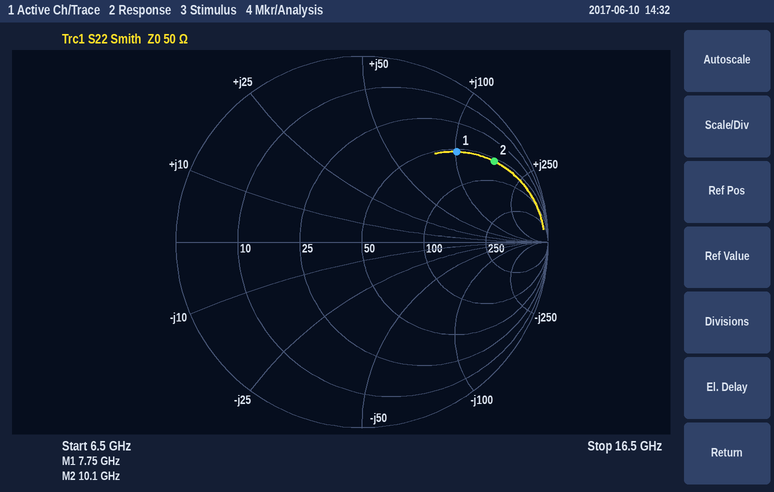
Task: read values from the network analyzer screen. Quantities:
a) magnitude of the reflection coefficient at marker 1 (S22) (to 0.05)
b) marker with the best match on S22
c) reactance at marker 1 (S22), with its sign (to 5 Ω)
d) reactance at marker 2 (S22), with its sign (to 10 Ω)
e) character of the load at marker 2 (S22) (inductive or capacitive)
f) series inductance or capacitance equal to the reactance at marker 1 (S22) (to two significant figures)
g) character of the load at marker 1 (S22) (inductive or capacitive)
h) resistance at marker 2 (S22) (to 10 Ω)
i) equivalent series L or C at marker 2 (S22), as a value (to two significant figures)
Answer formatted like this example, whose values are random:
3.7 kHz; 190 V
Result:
0.70; marker 1; +100 Ω; +160 Ω; inductive; 2.1 nH; inductive; 60 Ω; 2.5 nH
